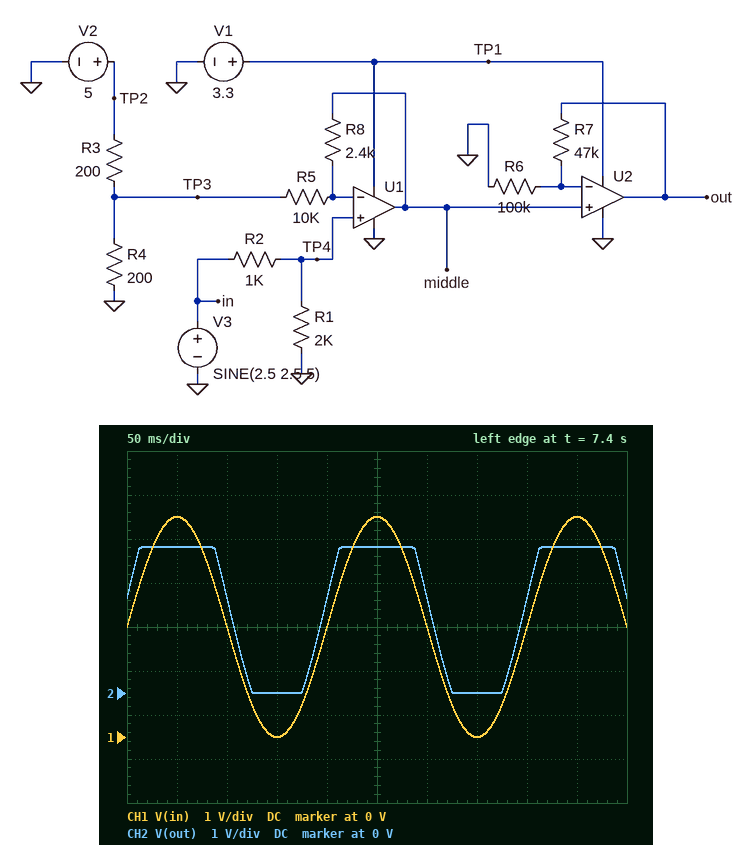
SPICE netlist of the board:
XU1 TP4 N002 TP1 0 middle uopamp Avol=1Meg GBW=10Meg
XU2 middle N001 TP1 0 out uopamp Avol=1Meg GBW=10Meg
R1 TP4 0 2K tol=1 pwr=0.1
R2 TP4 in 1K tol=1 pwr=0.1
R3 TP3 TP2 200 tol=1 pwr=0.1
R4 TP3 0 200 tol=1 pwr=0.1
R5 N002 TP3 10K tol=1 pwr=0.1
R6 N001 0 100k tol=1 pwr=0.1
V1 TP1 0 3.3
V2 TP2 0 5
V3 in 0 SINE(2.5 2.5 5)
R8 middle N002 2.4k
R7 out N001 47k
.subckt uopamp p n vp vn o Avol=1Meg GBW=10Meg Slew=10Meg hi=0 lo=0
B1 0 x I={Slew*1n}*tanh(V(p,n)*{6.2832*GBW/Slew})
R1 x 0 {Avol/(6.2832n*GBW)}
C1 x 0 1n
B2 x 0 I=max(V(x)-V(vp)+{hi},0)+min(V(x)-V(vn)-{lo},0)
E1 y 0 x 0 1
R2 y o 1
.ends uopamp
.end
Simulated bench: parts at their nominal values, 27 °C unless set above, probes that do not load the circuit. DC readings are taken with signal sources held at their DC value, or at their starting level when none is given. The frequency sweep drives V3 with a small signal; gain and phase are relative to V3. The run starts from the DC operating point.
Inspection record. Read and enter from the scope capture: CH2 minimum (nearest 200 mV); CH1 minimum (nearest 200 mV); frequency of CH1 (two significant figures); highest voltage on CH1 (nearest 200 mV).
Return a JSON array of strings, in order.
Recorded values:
["0 V", "0 V", "5.0 Hz", "5.0 V"]
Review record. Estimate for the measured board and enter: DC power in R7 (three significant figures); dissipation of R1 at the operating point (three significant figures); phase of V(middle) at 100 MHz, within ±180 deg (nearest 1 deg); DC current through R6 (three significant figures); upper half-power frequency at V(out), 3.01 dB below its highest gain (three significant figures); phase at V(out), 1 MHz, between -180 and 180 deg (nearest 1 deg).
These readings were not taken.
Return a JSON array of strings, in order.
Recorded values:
["10.1 µW", "1.39 mW", "-85 deg", "14.7 µA", "4.75 MHz", "-15 deg"]
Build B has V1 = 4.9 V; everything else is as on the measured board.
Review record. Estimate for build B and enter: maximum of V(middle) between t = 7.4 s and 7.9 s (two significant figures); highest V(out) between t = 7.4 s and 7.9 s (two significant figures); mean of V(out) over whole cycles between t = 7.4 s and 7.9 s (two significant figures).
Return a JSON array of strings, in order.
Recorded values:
["3.5 V", "4.9 V", "2.3 V"]
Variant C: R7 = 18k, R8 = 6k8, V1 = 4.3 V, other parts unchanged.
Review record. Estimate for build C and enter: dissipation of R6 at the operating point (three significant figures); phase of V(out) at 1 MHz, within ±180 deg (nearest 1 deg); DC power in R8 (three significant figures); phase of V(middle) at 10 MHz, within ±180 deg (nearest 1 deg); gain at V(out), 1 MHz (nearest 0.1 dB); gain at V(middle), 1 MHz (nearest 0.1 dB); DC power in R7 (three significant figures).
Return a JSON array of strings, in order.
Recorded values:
["12.2 µW", "-16 deg", "46.3 µW", "-59 deg", "2.2 dB", "0.8 dB", "2.20 µW"]
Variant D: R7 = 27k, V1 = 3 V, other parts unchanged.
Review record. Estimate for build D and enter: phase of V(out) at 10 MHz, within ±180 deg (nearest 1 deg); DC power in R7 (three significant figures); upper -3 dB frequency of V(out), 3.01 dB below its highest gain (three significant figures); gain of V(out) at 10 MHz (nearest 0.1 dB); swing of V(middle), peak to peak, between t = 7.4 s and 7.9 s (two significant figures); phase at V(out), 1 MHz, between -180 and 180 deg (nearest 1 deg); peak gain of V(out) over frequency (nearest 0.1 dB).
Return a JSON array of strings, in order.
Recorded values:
["-103 deg", "5.82 µW", "5.13 MHz", "-7.8 dB", "3.0 V", "-14 deg", "0.4 dB"]
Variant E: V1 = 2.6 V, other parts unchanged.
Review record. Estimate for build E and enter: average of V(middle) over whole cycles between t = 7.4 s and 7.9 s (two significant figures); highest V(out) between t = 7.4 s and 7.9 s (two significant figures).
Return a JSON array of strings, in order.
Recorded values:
["1.4 V", "2.6 V"]
